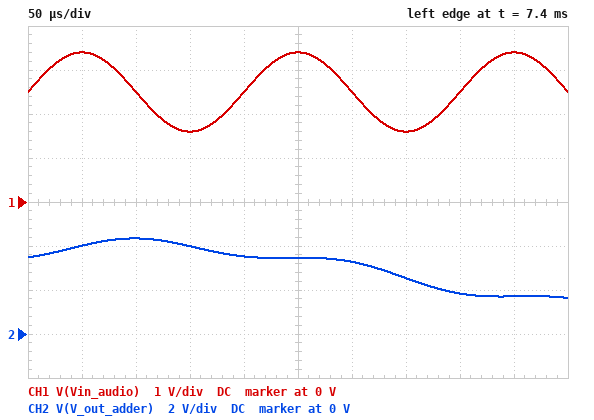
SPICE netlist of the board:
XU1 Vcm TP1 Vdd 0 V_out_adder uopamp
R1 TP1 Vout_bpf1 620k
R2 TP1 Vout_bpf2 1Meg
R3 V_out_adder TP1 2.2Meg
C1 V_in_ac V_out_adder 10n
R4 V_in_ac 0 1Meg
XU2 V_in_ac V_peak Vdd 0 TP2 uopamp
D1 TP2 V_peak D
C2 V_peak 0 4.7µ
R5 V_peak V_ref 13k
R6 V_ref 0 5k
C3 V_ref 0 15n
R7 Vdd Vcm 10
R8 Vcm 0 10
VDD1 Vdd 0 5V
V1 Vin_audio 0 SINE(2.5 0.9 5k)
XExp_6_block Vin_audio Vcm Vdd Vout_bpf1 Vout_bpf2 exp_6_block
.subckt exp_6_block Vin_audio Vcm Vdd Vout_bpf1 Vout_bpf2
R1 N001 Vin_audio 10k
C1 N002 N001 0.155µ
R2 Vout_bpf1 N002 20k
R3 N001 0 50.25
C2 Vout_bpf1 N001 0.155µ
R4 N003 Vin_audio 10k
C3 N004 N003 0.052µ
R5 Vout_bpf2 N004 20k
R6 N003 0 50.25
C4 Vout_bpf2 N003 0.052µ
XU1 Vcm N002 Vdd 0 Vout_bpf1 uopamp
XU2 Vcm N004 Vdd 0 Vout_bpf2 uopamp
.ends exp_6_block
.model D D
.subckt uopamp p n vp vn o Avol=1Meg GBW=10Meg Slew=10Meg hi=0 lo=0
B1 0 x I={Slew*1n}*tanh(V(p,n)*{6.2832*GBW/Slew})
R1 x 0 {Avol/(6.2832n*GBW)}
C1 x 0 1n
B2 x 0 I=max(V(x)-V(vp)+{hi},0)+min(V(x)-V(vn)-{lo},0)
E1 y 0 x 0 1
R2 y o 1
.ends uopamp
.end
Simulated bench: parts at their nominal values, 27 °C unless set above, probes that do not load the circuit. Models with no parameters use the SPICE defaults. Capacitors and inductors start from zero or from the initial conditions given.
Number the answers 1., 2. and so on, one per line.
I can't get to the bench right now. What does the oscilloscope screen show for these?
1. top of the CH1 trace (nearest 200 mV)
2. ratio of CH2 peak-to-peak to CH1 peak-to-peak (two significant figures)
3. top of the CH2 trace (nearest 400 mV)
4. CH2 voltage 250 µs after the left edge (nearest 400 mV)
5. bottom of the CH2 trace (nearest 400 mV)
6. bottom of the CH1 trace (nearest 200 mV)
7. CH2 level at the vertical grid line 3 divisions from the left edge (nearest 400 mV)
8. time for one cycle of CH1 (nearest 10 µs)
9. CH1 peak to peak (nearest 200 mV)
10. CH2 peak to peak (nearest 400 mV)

1. 3.4 V
2. 1.5
3. 4.4 V
4. 3.6 V
5. 1.6 V
6. 1.6 V
7. 4.0 V
8. 200 µs
9. 1.8 V
10. 2.8 V
